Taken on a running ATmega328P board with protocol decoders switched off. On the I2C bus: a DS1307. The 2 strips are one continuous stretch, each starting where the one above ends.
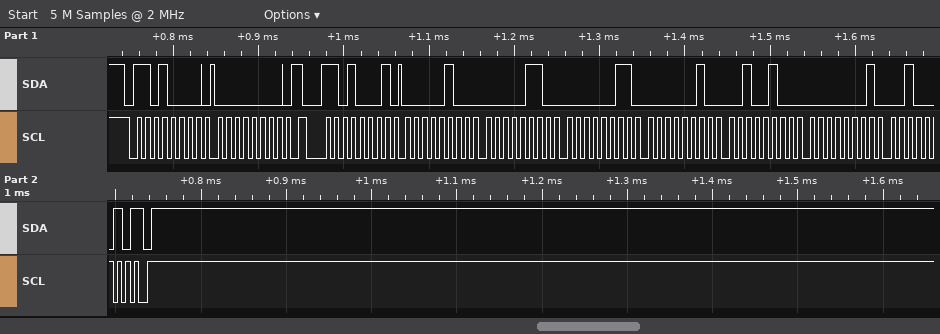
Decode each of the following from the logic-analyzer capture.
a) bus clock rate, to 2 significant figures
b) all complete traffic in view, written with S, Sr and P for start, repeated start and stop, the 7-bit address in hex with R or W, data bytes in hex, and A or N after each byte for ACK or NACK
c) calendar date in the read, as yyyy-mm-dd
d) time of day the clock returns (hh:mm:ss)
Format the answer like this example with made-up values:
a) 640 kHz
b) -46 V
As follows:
a) 100 kHz
b) S 68W A 00 A Sr 68R A 04 A 06 A 03 A 02 A 24 A 01 A 22 N P
c) 2022-01-24
d) 03:06:04
